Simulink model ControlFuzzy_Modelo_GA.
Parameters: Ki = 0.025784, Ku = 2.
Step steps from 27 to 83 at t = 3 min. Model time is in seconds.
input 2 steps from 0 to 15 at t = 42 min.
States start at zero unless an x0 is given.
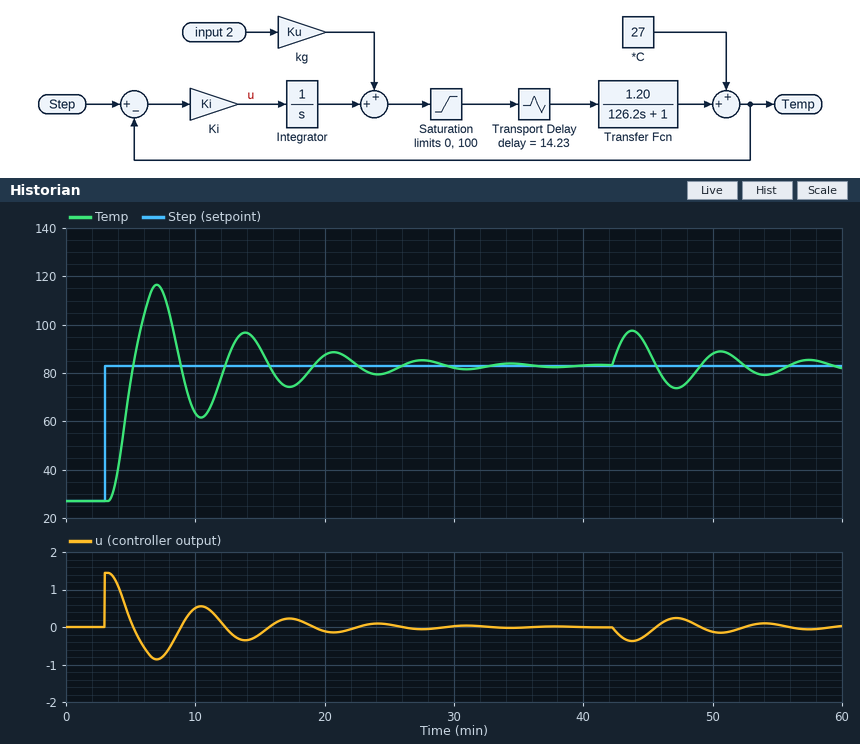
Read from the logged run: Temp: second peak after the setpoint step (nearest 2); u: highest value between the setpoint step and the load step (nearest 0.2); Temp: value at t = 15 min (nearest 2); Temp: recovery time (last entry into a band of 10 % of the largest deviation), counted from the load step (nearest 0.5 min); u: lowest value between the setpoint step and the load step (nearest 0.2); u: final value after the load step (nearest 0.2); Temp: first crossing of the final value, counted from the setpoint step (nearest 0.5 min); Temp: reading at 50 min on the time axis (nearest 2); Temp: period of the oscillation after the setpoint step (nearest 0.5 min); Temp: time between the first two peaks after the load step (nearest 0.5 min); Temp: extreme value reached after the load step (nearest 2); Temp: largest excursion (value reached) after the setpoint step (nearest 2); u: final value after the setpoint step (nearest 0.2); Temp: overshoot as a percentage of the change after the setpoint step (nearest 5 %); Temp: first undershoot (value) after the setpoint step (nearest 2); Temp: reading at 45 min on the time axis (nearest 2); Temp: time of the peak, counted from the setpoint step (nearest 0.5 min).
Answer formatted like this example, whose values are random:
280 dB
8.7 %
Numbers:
96
1.4
90
16.5 min
-0.8
0.0
2.0 min
88
7.0 min
7.0 min
98
116
0.0
60 %
62
90
4.0 min
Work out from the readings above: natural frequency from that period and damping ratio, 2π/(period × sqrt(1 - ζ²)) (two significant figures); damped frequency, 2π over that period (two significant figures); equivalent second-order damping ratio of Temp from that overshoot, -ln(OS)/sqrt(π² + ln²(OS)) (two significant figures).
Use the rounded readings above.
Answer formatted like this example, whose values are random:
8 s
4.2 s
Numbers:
0.91 rad/min
0.90 rad/min
0.16
